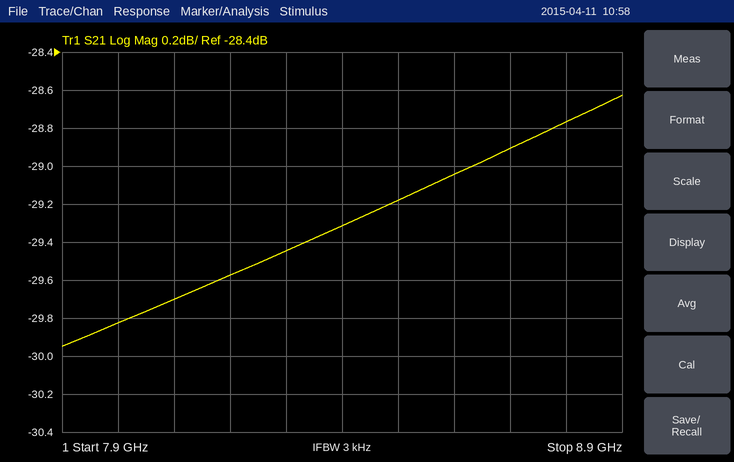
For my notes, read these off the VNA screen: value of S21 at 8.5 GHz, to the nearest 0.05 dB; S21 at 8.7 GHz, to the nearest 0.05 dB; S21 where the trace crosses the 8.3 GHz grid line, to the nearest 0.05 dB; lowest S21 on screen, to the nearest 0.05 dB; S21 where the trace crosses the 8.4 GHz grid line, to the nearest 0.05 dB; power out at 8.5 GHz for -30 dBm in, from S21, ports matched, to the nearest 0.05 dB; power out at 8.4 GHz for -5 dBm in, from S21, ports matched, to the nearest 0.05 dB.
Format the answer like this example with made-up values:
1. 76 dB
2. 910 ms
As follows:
1. -29.20 dB
2. -28.90 dB
3. -29.45 dB
4. -29.95 dB
5. -29.30 dB
6. -59.20 dBm
7. -34.30 dBm
